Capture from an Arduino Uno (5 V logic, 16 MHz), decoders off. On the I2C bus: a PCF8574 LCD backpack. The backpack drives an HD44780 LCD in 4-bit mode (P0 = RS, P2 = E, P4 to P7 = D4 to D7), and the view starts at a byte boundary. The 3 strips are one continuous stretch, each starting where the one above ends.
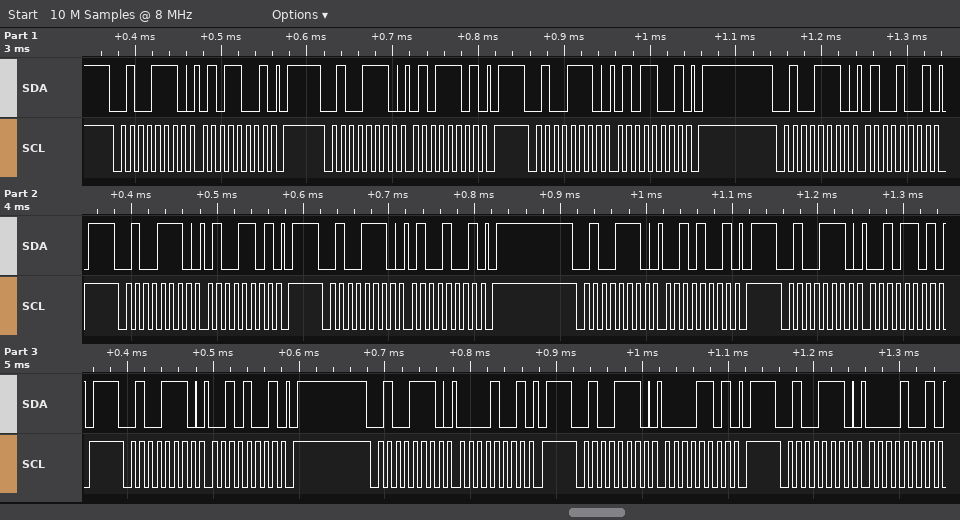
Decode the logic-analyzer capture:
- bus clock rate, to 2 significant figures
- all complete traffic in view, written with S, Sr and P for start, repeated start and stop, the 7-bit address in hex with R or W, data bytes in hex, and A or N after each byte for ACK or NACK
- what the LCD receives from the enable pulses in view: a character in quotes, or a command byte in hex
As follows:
100 kHz
S 27W A 59 A P S 27W A 5D A P S 27W A 59 A P S 27W A 49 A P S 27W A 4D A P S 27W A 49 A P S 27W A 29 A P S 27W A 2D A P S 27W A 29 A P S 27W A 09 A P S 27W A 0D A P S 27W A 09 A
'T' ' '
